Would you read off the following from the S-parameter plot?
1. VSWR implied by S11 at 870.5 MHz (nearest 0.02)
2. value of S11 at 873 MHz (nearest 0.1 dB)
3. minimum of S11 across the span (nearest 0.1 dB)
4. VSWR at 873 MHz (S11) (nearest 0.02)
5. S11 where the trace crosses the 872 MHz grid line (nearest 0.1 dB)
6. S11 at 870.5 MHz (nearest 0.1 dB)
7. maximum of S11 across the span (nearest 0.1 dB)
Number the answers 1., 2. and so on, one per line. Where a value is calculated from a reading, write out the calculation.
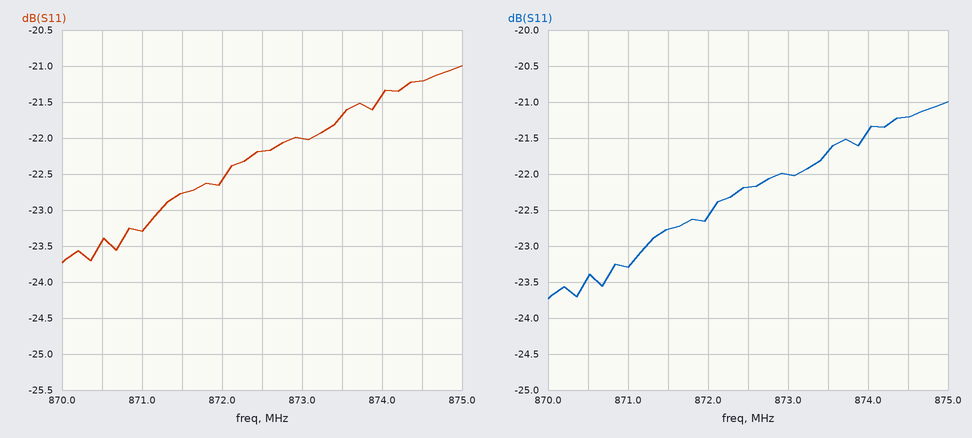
1. |Γ| = 10^(-23.4/20) = 0.0676; VSWR = (1 + 0.0676)/(1 − 0.0676) ≈ 1.15, so 1.14 to the nearest 0.02
2. -22.0 dB
3. -23.7 dB
4. |Γ| = 10^(-22/20) = 0.0794; VSWR = (1 + 0.0794)/(1 − 0.0794) ≈ 1.17, so 1.18 to the nearest 0.02
5. -22.6 dB
6. -23.4 dB
7. -21.0 dB
